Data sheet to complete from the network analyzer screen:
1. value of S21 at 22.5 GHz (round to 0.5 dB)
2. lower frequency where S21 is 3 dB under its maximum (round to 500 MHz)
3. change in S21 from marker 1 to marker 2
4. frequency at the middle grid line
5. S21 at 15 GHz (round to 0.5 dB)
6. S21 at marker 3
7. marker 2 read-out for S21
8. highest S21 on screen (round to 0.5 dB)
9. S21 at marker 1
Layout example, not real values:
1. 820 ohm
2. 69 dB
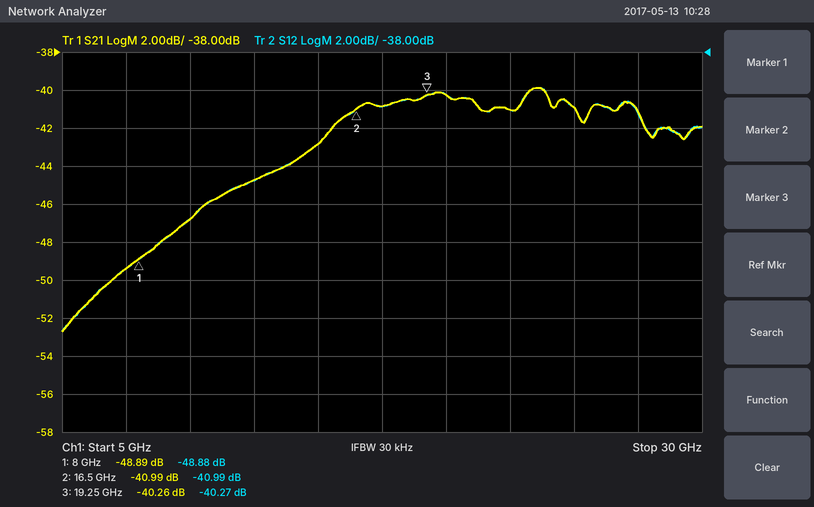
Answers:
1. -41.0 dB
2. 15.0 GHz
3. 7.90 dB
4. 17.5 GHz
5. -43.0 dB
6. -40.26 dB
7. -40.99 dB
8. -40.0 dB
9. -48.89 dB
